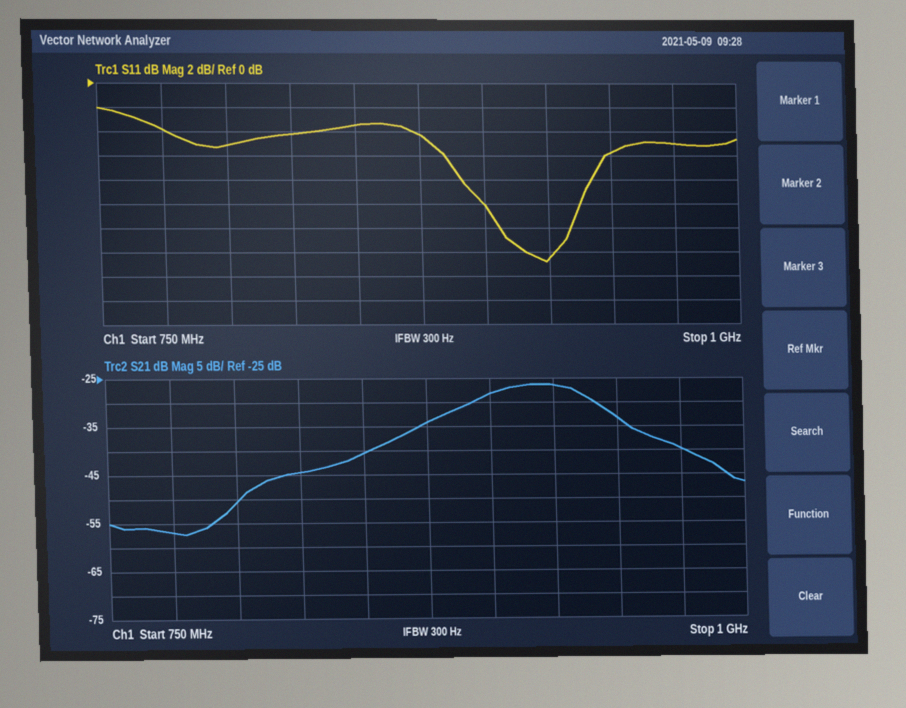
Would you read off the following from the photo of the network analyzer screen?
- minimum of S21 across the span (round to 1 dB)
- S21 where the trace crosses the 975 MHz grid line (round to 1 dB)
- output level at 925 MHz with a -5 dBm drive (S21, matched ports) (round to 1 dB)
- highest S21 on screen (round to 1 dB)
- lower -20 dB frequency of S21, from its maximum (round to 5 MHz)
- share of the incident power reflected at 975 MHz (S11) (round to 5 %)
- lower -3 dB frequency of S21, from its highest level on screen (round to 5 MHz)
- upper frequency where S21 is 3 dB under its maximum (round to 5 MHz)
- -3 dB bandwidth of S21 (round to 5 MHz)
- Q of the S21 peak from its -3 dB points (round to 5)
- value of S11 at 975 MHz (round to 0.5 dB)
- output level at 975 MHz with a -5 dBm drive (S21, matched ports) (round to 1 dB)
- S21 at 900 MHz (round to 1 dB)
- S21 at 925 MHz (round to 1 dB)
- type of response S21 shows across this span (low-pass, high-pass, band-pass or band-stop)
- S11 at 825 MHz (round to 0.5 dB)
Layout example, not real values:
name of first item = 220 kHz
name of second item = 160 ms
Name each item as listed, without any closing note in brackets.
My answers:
minimum of S21 across the span = -57 dB
S21 where the trace crosses the 975 MHz grid line = -40 dB
output level at 925 MHz with a -5 dBm drive (S21, matched ports) = -31 dBm
highest S21 on screen = -26 dB
lower -20 dB frequency of S21, from its maximum = 810 MHz
share of the incident power reflected at 975 MHz (S11) = 30 %
lower -3 dB frequency of S21, from its highest level on screen = 895 MHz
upper frequency where S21 is 3 dB under its maximum = 940 MHz
-3 dB bandwidth of S21 = 45 MHz
Q of the S21 peak from its -3 dB points = 20
value of S11 at 975 MHz = -5.0 dB
output level at 975 MHz with a -5 dBm drive (S21, matched ports) = -45 dBm
S21 at 900 MHz = -28 dB
S21 at 925 MHz = -26 dB
type of response S21 shows across this span = band-pass
S11 at 825 MHz = -4.0 dB
